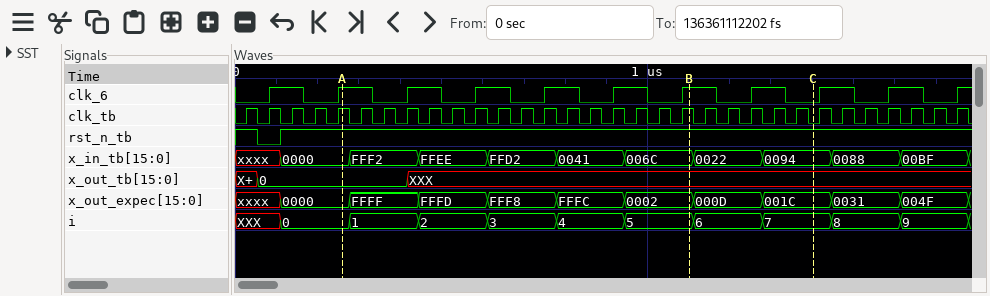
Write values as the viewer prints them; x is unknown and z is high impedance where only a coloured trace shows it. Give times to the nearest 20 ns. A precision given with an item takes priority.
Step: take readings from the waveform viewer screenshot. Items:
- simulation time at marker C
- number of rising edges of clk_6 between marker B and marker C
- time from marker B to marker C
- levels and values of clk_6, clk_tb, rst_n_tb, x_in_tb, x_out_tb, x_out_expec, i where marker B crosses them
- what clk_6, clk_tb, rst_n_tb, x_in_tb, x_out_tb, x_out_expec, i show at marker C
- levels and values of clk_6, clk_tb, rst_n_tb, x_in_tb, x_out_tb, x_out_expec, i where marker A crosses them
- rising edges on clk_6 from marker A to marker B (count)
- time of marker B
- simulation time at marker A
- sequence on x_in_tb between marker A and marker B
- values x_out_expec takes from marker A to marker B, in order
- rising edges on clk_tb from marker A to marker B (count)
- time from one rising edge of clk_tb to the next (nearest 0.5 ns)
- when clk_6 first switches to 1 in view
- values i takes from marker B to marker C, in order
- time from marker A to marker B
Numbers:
1400 ns
1
300 ns
clk_6=1, clk_tb=1, rst_n_tb=1, x_in_tb=006C, x_out_tb=XXX, x_out_expec=0002, i=5
clk_6=0, clk_tb=0, rst_n_tb=1, x_in_tb=0094, x_out_tb=XXX, x_out_expec=001C, i=7
clk_6=1, clk_tb=1, rst_n_tb=1, x_in_tb=0000, x_out_tb=0, x_out_expec=0000, i=0
5
1100 ns
260 ns
0000, FFF2, FFEE, FFD2, 0041, 006C
0000, FFFF, FFFD, FFF8, FFFC, 0002
15
55.5 ns
80 ns
5, 6, 7
840 ns
